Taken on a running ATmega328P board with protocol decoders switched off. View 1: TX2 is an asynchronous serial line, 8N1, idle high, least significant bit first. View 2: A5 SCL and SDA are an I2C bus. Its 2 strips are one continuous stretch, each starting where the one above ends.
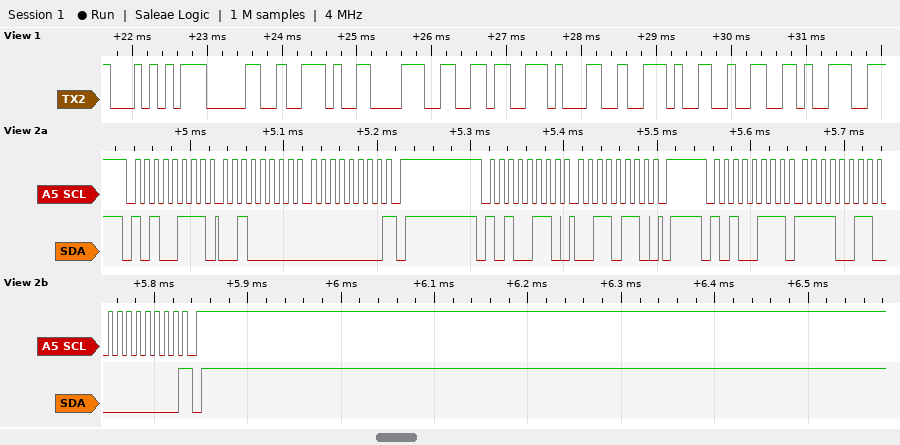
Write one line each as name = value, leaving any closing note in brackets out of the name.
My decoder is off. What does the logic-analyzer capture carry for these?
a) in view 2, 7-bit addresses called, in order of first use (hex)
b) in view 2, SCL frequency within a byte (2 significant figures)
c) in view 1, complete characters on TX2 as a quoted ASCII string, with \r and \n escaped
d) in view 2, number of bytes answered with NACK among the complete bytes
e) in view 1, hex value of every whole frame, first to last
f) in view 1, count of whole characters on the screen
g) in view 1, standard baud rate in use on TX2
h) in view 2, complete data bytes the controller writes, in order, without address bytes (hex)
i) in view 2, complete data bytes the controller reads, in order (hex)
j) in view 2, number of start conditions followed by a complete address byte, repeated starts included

in view 2, 7-bit addresses called, in order of first use = 0x53
in view 2, SCL frequency within a byte = 100 kHz
in view 1, complete characters on TX2 as a quoted ASCII string, with \r and \n escaped = "T0.861.29"
in view 2, number of bytes answered with NACK among the complete bytes = 2
in view 1, hex value of every whole frame, first to last = 54 30 2E 38 36 31 2E 32 39
in view 1, count of whole characters on the screen = 9
in view 1, standard baud rate in use on TX2 = 9600 baud
in view 2, complete data bytes the controller writes, in order, without address bytes = 36
in view 2, complete data bytes the controller reads, in order = 20 00 F3 00
in view 2, number of start conditions followed by a complete address byte, repeated starts included = 3
